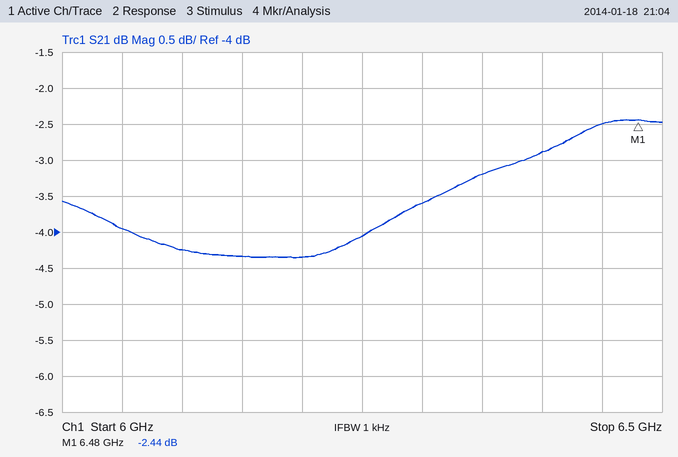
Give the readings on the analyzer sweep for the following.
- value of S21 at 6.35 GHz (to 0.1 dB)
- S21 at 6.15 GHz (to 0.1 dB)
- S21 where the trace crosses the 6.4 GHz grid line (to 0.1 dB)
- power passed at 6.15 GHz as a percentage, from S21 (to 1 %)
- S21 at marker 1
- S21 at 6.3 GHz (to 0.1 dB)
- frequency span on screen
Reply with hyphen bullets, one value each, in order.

- -3.2 dB
- -4.3 dB
- -2.9 dB
- 37 %
- -2.44 dB
- -3.6 dB
- 500 MHz
